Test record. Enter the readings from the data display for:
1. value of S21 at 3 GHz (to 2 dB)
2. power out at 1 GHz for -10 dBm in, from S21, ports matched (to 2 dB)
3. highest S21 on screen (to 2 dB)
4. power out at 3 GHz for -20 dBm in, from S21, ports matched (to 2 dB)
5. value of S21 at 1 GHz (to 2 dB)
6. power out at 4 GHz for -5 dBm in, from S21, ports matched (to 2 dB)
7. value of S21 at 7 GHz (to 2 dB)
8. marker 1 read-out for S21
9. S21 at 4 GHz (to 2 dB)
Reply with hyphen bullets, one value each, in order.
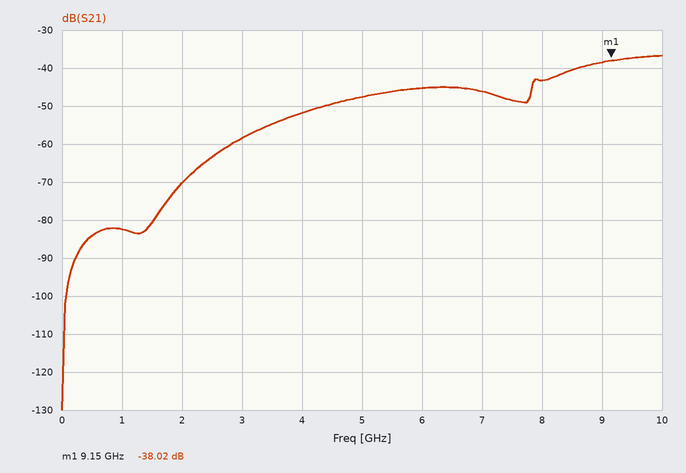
- -58 dB
- -92 dBm
- -36 dB
- -78 dBm
- -82 dB
- -56 dBm
- -46 dB
- -38.02 dB
- -52 dB
